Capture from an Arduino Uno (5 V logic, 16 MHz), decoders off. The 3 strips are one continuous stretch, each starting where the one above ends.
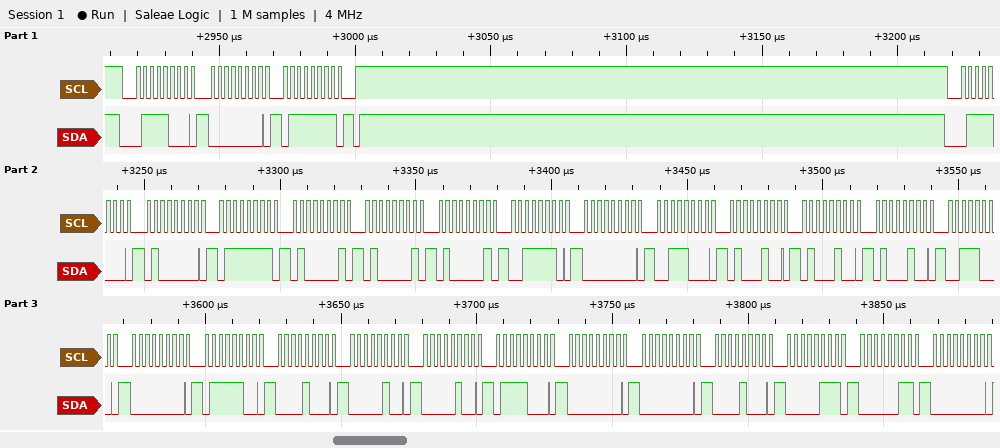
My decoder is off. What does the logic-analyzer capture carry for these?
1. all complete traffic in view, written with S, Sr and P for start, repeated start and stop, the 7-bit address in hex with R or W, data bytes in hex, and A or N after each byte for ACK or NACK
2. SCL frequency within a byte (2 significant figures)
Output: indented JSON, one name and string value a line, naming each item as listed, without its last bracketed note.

{
  "all complete traffic in view, written with S, Sr and P for start, repeated start and stop, the 7-bit address in hex with R or W, data bytes in hex, and A or N after each byte for ACK or NACK": "S 3CW A 00 A 7F A P S 3CW A 40 A 7F A 41 A 41 A 41 A 3E A 00 A 38 A 44 A 44 A 44 A 38 A 00 A 7C A 08 A 04 A 04 A 78 A 00 A 00 A 08 A 07 A 03 A 00 A",
  "SCL frequency within a byte": "400 kHz"
}
